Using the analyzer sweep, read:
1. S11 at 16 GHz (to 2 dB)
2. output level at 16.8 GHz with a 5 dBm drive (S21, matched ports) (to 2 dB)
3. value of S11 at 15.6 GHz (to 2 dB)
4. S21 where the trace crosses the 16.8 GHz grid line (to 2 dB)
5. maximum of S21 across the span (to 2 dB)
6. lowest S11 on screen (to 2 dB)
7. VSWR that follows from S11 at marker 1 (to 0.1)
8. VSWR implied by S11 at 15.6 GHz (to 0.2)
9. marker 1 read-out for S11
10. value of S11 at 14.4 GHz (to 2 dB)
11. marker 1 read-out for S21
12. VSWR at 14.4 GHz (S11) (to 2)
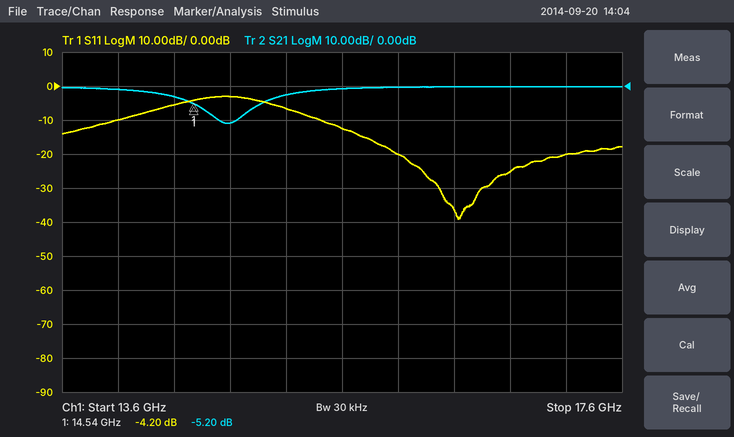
-20 dB
4 dBm
-12 dB
0 dB
0 dB
-40 dB
4.2
1.6
-4.20 dB
-6 dB
-5.20 dB
4
